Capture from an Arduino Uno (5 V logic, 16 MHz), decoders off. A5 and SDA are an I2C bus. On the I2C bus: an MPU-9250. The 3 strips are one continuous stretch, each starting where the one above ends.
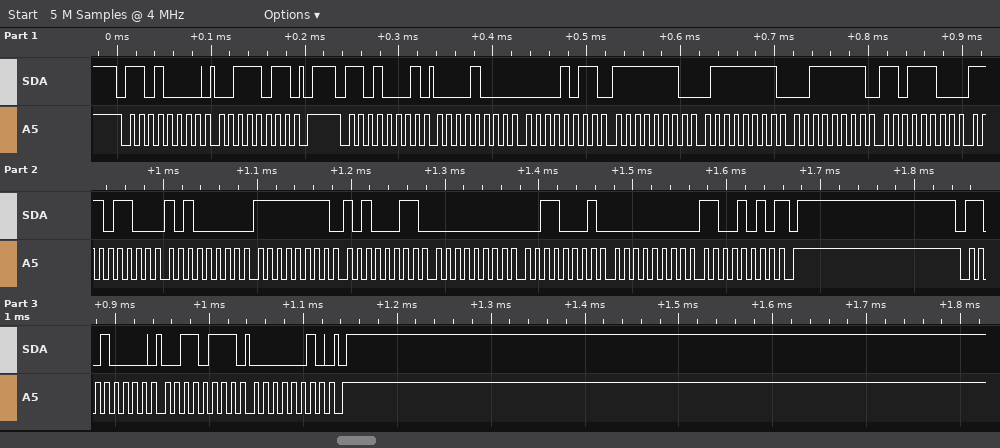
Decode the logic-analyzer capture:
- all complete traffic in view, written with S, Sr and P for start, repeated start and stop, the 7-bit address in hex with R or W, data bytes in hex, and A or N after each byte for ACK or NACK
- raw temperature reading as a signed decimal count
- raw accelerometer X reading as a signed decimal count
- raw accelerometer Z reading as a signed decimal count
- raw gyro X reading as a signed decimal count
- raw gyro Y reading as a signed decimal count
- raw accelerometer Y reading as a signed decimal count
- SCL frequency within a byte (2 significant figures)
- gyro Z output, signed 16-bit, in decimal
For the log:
S 68W A 3B A P S 68R A 08 A 0B A FE A 7F A 3F A DC A EC A A0 A FF A A3 A 00 A 31 A 00 A CA N P S 68W A 37 A 02 A P
-4960
2059
16348
-93
49
-385
100 kHz
202
